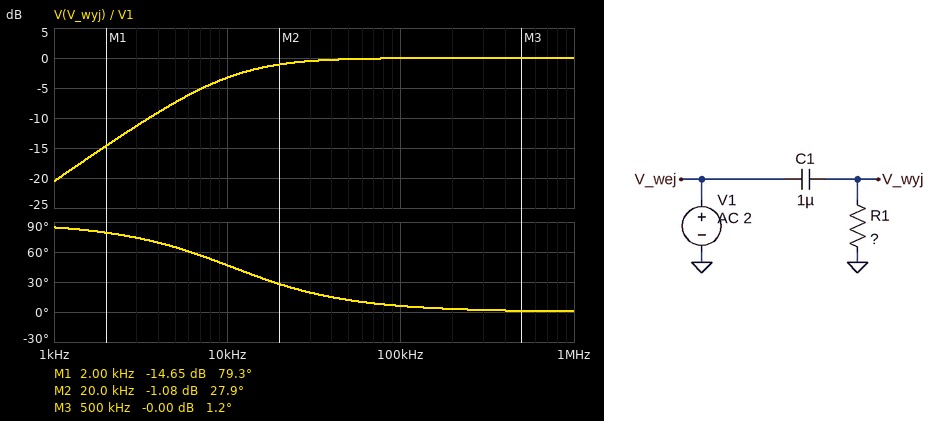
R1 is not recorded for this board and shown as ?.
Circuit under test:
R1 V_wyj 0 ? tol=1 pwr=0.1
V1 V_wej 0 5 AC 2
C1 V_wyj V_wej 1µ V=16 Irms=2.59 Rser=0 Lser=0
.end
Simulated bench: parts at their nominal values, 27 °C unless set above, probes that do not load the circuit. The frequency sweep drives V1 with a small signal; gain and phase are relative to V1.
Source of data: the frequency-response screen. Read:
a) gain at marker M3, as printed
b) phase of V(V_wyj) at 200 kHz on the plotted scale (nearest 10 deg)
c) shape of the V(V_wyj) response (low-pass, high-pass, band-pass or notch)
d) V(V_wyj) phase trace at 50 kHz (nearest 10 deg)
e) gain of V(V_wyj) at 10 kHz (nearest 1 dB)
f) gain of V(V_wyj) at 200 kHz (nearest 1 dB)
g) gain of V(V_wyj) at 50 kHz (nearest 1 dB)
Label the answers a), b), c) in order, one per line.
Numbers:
a) -0.00 dB
b) 0 deg
c) high-pass
d) 10 deg
e) -3 dB
f) 0 dB
g) 0 dB
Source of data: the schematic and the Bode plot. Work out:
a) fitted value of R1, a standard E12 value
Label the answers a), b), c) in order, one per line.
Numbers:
a) 15 Ω
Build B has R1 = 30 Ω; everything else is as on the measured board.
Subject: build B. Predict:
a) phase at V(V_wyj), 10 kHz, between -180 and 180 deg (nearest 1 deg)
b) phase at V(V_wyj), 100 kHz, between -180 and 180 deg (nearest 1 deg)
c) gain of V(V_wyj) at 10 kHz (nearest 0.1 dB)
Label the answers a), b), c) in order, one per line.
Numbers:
a) 28 deg
b) 3 deg
c) -1.1 dB
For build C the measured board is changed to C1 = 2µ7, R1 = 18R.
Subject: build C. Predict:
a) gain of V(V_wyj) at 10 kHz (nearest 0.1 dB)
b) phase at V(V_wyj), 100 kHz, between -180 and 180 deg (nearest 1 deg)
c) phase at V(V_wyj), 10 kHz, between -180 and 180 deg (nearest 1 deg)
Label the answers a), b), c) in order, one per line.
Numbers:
a) -0.4 dB
b) 2 deg
c) 18 deg
